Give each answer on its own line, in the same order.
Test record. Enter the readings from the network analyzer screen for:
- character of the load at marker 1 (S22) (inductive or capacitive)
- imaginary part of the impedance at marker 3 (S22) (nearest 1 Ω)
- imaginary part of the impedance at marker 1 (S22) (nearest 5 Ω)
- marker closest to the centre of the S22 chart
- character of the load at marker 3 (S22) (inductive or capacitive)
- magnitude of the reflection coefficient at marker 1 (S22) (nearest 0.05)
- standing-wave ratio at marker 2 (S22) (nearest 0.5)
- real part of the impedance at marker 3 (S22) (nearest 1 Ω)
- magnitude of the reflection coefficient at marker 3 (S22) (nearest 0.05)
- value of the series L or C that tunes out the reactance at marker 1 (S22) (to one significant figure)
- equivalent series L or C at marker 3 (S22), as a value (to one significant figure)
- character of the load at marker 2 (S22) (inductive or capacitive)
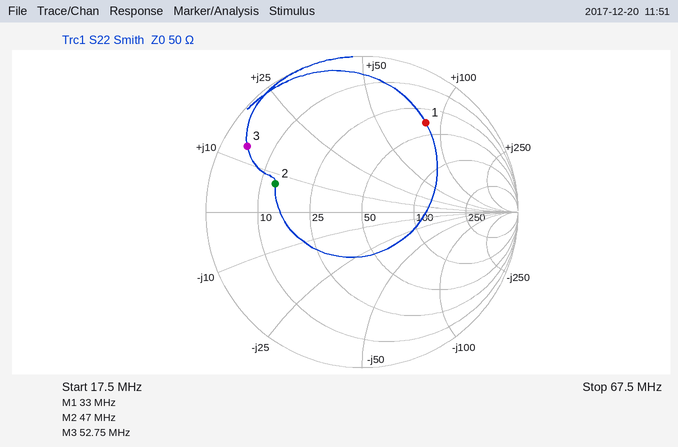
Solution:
inductive
+13 Ω
+85 Ω
marker 2
inductive
0.70
4.0
4 Ω
0.85
60 pF
40 nH
inductive
